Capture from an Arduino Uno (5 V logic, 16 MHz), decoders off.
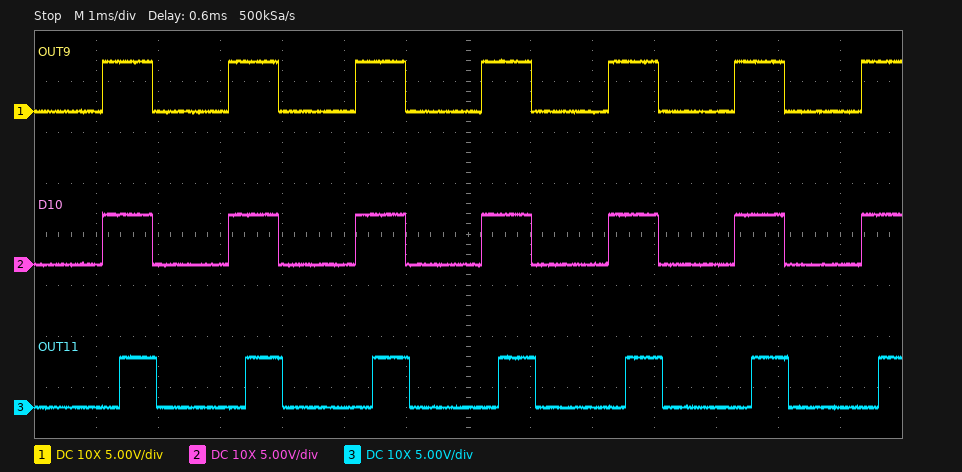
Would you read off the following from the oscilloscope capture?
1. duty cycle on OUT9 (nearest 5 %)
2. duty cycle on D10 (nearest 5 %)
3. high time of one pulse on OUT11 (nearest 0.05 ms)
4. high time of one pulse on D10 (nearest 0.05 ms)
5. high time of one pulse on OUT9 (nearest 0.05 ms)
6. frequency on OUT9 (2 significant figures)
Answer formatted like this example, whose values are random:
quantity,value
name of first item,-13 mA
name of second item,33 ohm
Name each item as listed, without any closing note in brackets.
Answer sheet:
quantity,value
duty cycle on OUT9,40 %
duty cycle on D10,40 %
high time of one pulse on OUT11,0.60 ms
high time of one pulse on D10,0.80 ms
high time of one pulse on OUT9,0.80 ms
frequency on OUT9,490 Hz
